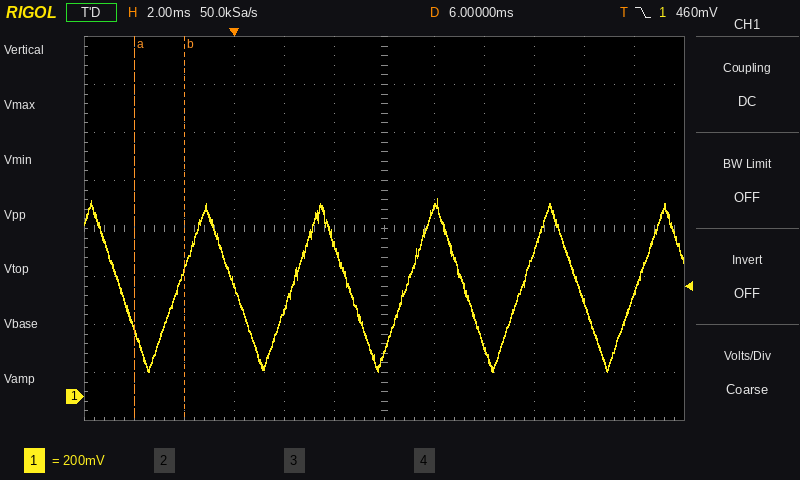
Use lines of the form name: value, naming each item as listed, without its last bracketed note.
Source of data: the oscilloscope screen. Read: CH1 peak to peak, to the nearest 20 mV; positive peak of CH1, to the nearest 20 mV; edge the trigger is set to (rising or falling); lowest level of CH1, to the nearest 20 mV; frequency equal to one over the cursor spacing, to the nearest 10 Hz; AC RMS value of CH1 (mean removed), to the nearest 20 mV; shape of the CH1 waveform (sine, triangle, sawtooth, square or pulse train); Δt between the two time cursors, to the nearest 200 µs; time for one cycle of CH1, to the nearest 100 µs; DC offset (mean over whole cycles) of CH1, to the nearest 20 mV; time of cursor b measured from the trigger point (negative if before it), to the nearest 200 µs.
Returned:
CH1 peak to peak, to the nearest 20 mV: 720 mV
positive peak of CH1, to the nearest 20 mV: 820 mV
edge the trigger is set to: falling
lowest level of CH1, to the nearest 20 mV: 100 mV
frequency equal to one over the cursor spacing, to the nearest 10 Hz: 500 Hz
AC RMS value of CH1 (mean removed), to the nearest 20 mV: 200 mV
shape of the CH1 waveform: triangle
Δt between the two time cursors, to the nearest 200 µs: 2.0 ms
time for one cycle of CH1, to the nearest 100 µs: 4.6 ms
DC offset (mean over whole cycles) of CH1, to the nearest 20 mV: 460 mV
time of cursor b measured from the trigger point (negative if before it), to the nearest 200 µs: -2.0 ms
